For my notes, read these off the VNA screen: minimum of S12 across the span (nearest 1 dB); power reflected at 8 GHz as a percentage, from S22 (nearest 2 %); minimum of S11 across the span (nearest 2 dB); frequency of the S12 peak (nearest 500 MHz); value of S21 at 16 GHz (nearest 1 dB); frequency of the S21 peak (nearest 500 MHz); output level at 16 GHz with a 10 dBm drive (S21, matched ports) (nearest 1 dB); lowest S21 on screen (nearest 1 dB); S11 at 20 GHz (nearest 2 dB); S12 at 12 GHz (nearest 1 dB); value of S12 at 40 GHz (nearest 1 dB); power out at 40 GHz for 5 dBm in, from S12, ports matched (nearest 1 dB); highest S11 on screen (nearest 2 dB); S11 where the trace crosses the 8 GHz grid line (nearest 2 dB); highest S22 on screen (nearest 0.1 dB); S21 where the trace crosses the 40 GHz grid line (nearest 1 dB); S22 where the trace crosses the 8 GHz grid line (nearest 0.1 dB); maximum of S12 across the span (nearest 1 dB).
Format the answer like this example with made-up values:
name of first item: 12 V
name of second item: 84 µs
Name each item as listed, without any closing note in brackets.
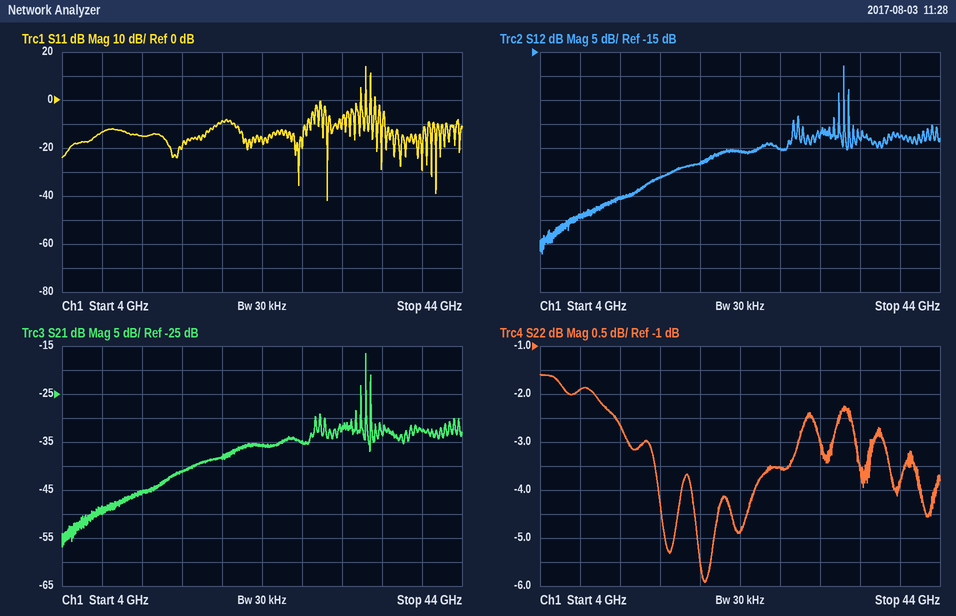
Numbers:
minimum of S12 across the span: -57 dB
power reflected at 8 GHz as a percentage, from S22: 64 %
minimum of S11 across the span: -42 dB
frequency of the S12 peak: 34.5 GHz
value of S21 at 16 GHz: -41 dB
frequency of the S21 peak: 34.5 GHz
output level at 16 GHz with a 10 dBm drive (S21, matched ports): -31 dBm
lowest S21 on screen: -57 dB
S11 at 20 GHz: -8 dB
S12 at 12 GHz: -45 dB
value of S12 at 40 GHz: -33 dB
power out at 40 GHz for 5 dBm in, from S12, ports matched: -28 dBm
highest S11 on screen: 14 dB
S11 where the trace crosses the 8 GHz grid line: -14 dB
highest S22 on screen: -1.6 dB
S21 where the trace crosses the 40 GHz grid line: -33 dB
S22 where the trace crosses the 8 GHz grid line: -1.9 dB
maximum of S12 across the span: -18 dB
